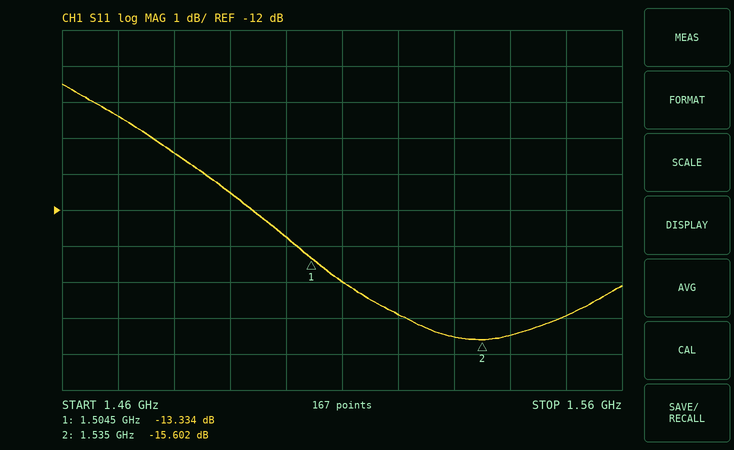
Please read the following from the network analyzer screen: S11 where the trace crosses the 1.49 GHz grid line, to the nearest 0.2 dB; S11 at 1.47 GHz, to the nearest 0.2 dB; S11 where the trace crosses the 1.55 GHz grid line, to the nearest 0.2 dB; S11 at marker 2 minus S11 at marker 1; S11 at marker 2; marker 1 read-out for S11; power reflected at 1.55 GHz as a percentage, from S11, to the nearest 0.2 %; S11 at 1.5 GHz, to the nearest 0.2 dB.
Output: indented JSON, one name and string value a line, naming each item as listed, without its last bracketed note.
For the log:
{
  "S11 where the trace crosses the 1.49 GHz grid line, to the nearest 0.2 dB": "-11.6 dB",
  "S11 at 1.47 GHz, to the nearest 0.2 dB": "-9.4 dB",
  "S11 where the trace crosses the 1.55 GHz grid line, to the nearest 0.2 dB": "-15.0 dB",
  "S11 at marker 2 minus S11 at marker 1": "-2.268 dB",
  "S11 at marker 2": "-15.602 dB",
  "marker 1 read-out for S11": "-13.334 dB",
  "power reflected at 1.55 GHz as a percentage, from S11, to the nearest 0.2 %": "3.2 %",
  "S11 at 1.5 GHz, to the nearest 0.2 dB": "-12.8 dB"
}
